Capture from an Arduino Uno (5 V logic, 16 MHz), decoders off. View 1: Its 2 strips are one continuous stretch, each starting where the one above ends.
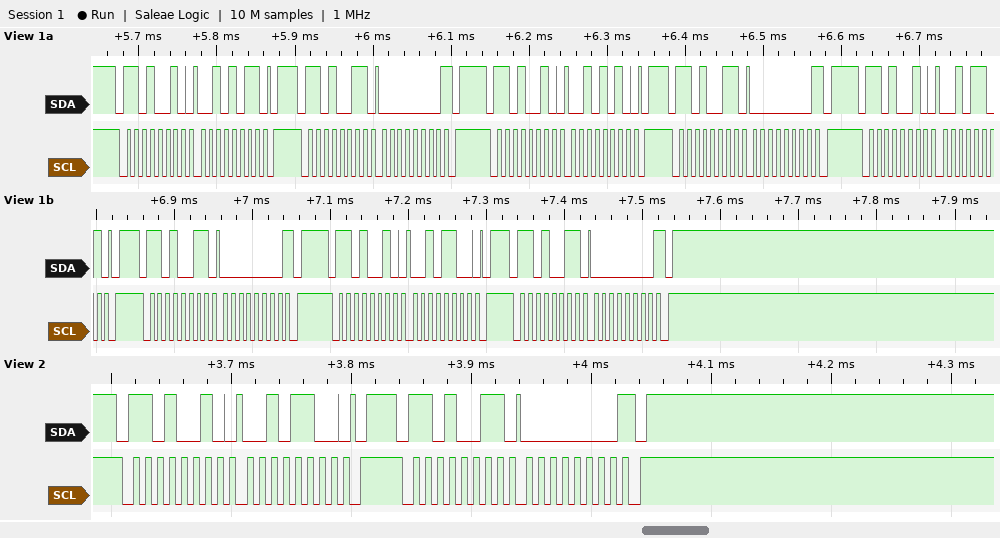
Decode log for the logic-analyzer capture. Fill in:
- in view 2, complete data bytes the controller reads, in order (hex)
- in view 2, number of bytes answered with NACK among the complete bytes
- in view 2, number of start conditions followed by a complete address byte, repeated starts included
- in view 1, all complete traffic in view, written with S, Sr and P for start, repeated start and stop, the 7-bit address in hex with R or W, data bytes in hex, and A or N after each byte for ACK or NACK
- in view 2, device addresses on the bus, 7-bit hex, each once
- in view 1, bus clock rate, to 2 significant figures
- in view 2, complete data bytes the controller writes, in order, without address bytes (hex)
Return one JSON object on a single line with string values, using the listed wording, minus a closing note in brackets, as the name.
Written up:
{"in view 2, complete data bytes the controller reads, in order": "00", "in view 2, number of bytes answered with NACK among the complete bytes": "1", "in view 2, number of start conditions followed by a complete address byte, repeated starts included": "2", "in view 1, all complete traffic in view, written with S, Sr and P for start, repeated start and stop, the 7-bit address in hex with R or W, data bytes in hex, and A or N after each byte for ACK or NACK": "S 69W A 2B A P S 69R A 00 N P S 69W A 2A A P S 69R A 00 N P S 69W A 2D A P S 69R A 00 N P S 69W A 2C A P S 69R A 00 N P", "in view 2, device addresses on the bus, 7-bit hex, each once": "0x69", "in view 1, bus clock rate, to 2 significant figures": "100 kHz", "in view 2, complete data bytes the controller writes, in order, without address bytes": "2C"}
